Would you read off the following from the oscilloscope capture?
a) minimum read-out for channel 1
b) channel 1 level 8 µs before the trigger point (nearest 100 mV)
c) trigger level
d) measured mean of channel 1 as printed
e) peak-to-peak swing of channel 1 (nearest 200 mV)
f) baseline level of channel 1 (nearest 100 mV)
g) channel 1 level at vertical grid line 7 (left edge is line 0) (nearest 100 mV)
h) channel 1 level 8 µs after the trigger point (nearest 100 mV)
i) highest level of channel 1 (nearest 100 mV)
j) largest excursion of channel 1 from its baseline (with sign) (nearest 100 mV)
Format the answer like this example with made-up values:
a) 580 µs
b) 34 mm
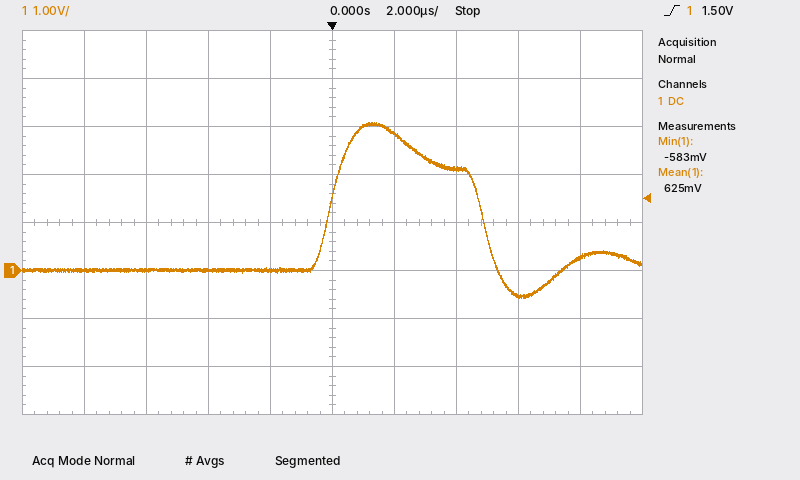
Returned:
a) -583 mV
b) 0.0 V
c) 1.50 V
d) 625 mV
e) 3.6 V
f) 0.0 V
g) 2.1 V
h) 300 mV
i) 3.1 V
j) +3.1 V
